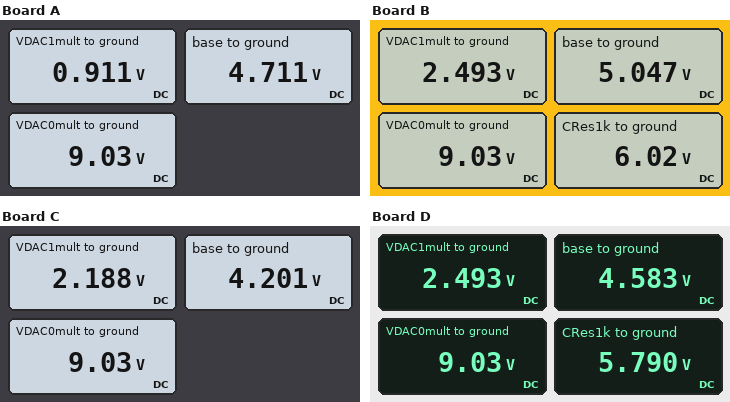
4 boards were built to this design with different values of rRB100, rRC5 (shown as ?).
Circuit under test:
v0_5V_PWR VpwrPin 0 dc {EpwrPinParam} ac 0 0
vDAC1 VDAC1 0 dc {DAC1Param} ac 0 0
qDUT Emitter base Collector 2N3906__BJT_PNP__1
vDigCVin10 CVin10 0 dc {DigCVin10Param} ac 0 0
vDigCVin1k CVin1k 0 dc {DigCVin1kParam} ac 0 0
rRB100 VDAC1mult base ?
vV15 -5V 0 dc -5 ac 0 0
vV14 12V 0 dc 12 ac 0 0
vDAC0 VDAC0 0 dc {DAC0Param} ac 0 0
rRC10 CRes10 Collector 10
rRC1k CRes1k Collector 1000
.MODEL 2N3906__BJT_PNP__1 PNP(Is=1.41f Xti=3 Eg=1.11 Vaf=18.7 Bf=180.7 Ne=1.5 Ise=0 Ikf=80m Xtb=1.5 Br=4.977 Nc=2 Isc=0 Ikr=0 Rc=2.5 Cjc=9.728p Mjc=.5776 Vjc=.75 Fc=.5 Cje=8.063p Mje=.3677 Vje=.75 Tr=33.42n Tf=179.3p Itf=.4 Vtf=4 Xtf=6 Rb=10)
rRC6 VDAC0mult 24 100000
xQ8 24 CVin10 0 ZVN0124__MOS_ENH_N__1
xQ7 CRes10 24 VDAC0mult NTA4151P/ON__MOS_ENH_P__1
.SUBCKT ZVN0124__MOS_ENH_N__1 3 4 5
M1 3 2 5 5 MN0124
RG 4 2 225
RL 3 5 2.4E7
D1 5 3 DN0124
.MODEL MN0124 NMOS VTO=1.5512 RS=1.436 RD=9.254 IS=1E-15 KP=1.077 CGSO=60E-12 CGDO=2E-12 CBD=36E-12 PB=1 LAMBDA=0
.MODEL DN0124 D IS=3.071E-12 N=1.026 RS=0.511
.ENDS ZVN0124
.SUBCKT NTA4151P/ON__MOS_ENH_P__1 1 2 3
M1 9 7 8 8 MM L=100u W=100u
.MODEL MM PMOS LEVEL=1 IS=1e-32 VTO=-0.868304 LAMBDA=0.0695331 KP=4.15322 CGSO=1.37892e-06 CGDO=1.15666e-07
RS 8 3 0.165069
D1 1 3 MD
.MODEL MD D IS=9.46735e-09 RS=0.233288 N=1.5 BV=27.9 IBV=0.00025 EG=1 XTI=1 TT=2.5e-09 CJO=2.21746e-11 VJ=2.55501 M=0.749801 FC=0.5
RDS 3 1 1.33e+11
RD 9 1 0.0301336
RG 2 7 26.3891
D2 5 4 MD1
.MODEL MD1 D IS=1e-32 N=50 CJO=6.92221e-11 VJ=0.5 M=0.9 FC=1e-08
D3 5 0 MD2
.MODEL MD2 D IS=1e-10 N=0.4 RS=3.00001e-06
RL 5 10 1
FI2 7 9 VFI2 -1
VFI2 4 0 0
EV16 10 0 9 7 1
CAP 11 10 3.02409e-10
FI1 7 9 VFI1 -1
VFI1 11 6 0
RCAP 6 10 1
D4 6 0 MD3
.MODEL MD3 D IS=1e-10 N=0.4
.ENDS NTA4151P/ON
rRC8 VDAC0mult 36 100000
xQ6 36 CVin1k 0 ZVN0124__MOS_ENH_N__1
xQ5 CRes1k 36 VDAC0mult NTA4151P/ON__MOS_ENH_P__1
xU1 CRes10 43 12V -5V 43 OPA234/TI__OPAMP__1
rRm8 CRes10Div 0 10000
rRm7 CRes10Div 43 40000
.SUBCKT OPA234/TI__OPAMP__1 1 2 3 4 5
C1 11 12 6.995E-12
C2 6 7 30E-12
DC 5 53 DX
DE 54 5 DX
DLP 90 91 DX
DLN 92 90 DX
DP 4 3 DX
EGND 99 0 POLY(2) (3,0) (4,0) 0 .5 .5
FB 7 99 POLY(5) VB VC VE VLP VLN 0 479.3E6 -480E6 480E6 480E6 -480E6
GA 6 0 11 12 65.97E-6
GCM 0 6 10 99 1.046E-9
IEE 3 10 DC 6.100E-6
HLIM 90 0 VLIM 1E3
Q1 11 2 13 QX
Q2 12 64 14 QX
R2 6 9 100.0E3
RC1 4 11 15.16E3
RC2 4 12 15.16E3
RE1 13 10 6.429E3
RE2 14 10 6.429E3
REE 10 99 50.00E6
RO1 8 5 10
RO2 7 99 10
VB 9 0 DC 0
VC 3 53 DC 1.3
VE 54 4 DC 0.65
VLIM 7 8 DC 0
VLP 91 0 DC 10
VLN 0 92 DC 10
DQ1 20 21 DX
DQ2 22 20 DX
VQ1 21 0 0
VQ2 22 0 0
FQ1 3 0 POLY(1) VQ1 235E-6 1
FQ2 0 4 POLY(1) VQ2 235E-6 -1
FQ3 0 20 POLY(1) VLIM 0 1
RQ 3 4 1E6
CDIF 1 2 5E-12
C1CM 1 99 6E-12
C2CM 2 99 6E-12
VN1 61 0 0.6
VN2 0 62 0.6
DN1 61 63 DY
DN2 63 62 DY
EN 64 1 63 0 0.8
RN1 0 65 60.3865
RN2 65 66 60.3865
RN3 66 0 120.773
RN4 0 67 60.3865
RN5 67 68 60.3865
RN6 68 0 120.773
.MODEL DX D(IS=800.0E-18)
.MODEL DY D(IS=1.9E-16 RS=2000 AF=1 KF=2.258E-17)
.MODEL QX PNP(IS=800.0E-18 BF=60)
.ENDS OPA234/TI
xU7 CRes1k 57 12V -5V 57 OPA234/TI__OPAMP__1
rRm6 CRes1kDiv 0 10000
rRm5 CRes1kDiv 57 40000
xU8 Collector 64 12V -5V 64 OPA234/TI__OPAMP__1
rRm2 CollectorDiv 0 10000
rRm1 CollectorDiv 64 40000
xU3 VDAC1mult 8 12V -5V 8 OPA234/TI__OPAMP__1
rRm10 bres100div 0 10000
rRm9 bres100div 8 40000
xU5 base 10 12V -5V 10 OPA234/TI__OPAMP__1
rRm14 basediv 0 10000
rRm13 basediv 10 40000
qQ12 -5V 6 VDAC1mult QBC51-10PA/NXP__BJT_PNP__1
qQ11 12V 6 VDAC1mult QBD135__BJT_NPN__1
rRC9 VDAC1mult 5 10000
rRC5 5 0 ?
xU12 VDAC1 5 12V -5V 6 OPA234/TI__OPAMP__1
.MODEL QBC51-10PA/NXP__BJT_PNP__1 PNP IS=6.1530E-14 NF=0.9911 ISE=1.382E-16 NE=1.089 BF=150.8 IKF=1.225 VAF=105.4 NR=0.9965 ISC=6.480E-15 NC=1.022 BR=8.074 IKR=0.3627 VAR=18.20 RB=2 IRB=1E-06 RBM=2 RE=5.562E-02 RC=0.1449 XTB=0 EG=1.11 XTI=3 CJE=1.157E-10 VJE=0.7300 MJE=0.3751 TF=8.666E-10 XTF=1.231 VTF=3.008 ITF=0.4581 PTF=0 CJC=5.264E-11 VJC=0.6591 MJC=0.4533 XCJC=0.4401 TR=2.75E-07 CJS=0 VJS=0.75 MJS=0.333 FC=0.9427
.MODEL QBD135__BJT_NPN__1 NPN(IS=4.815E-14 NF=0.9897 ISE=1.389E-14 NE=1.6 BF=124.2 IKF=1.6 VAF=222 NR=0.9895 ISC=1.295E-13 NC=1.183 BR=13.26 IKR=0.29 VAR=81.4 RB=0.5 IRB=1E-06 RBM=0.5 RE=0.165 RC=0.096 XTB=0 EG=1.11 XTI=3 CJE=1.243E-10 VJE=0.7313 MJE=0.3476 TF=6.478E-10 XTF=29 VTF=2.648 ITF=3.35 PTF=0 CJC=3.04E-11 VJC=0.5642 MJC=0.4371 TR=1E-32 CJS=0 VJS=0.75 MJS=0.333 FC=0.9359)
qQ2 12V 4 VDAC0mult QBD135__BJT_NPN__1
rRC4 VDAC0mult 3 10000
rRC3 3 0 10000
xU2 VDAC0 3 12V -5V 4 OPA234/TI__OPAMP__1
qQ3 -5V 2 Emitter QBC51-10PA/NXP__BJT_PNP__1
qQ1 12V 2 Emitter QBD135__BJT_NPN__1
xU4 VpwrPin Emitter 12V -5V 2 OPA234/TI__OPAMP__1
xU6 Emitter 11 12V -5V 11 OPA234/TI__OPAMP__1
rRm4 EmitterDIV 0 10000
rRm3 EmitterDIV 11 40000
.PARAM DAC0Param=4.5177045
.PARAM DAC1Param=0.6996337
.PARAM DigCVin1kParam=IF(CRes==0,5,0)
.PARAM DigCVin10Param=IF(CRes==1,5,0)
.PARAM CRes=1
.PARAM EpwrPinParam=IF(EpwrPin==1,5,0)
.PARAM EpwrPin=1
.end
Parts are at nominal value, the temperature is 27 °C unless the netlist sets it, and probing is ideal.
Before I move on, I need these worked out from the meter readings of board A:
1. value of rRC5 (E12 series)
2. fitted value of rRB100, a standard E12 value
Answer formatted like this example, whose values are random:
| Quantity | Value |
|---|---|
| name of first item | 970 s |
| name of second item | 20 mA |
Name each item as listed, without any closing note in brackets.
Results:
| Quantity | Value |
|---|---|
| value of rRC5 | 33 kΩ |
| fitted value of rRB100, a standard E12 value | 180 Ω |
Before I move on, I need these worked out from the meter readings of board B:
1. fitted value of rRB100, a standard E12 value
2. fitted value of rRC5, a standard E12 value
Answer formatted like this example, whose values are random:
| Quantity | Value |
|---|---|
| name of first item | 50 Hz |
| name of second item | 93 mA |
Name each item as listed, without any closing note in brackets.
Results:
| Quantity | Value |
|---|---|
| fitted value of rRB100, a standard E12 value | 330 Ω |
| fitted value of rRC5, a standard E12 value | 3.9 kΩ |
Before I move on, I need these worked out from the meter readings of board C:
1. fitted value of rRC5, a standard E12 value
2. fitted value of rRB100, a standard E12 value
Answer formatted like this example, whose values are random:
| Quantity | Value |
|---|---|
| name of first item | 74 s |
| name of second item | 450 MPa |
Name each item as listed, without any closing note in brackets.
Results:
| Quantity | Value |
|---|---|
| fitted value of rRC5, a standard E12 value | 4.7 kΩ |
| fitted value of rRB100, a standard E12 value | 33 Ω |
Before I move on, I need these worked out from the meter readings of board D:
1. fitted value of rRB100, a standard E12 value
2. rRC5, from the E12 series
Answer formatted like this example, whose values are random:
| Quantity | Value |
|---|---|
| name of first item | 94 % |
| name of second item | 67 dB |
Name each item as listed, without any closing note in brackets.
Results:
| Quantity | Value |
|---|---|
| fitted value of rRB100, a standard E12 value | 68 Ω |
| rRC5, from the E12 series | 3.9 kΩ |
